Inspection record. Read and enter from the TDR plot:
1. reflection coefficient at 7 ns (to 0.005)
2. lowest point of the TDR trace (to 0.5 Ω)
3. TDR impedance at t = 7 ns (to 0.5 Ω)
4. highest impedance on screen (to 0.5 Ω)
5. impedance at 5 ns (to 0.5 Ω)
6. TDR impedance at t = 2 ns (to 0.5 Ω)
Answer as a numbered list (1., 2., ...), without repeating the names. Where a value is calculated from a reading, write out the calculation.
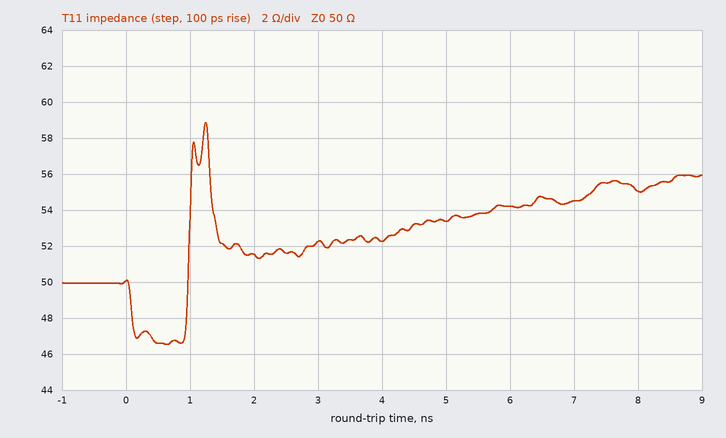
1. (54.5 − 50)/(54.5 + 50) ≈ +0.0431, so +0.045 to the nearest 0.005
2. 46.5 Ω
3. 54.5 Ω
4. 59.0 Ω
5. 53.5 Ω
6. 51.5 Ω
